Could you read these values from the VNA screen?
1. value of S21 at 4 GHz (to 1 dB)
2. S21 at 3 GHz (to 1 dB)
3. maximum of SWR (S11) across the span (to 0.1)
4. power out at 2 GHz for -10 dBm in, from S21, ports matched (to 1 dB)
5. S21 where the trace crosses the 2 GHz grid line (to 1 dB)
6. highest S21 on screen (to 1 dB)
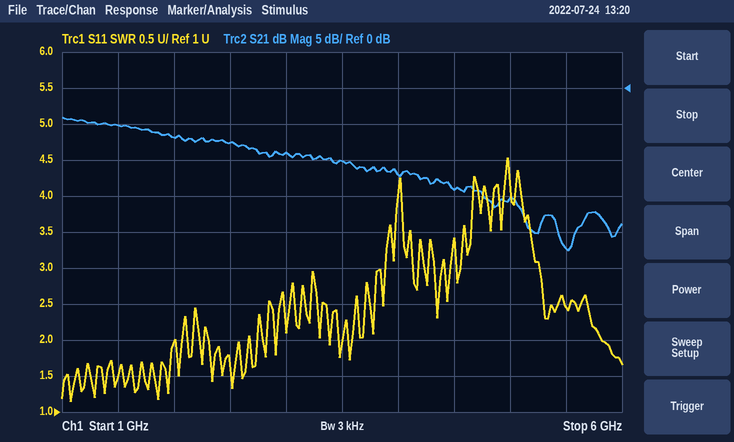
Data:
-12 dB
-9 dB
4.5
-17 dBm
-7 dB
-4 dB
